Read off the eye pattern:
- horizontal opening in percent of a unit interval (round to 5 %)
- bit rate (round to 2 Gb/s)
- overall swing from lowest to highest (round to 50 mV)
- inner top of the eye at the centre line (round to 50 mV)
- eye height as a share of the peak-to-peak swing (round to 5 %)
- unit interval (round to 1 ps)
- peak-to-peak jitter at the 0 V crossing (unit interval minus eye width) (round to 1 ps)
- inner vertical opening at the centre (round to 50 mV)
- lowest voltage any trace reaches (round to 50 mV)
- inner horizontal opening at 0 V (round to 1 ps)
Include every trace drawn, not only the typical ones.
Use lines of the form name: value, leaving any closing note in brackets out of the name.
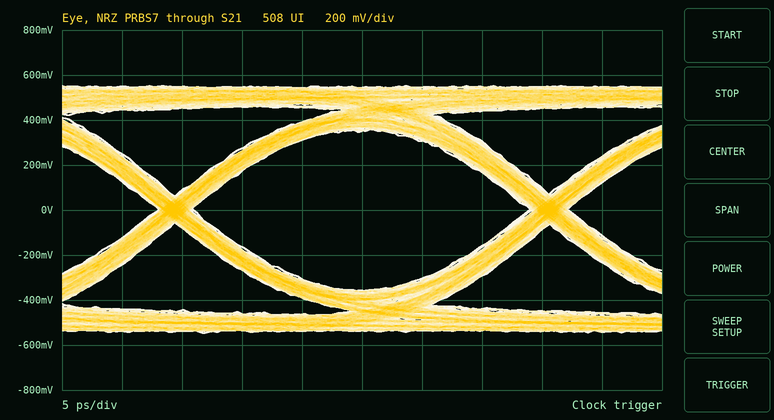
horizontal opening in percent of a unit interval: 90 %
bit rate: 32 Gb/s
overall swing from lowest to highest: 1.10 V
inner top of the eye at the centre line: 350 mV
eye height as a share of the peak-to-peak swing: 65 %
unit interval: 31 ps
peak-to-peak jitter at the 0 V crossing (unit interval minus eye width): 3 ps
inner vertical opening at the centre: 700 mV
lowest voltage any trace reaches: -550 mV
inner horizontal opening at 0 V: 28 ps
